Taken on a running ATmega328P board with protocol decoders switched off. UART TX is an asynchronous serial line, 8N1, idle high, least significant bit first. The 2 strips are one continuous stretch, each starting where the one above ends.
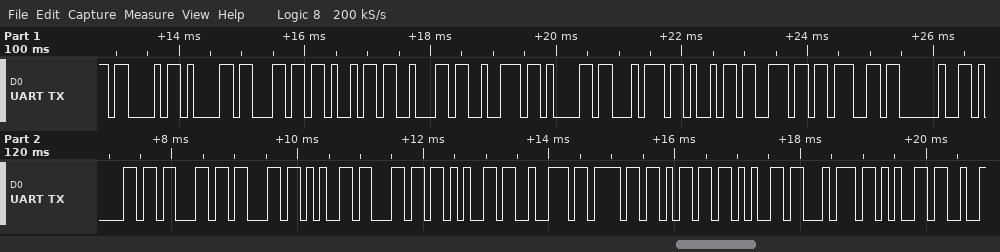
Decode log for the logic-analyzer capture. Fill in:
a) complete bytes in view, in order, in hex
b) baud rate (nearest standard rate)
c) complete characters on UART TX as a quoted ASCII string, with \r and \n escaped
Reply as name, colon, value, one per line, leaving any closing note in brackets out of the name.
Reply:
complete bytes in view, in order, in hex: 43 61 6C 69 62 72 61 74 69 6E 67 20 61 63 63 65 6C 65 72 6F 6D 65 74 65
baud rate: 9600 baud
complete characters on UART TX as a quoted ASCII string, with \r and \n escaped: "Calibrating acceleromete"
